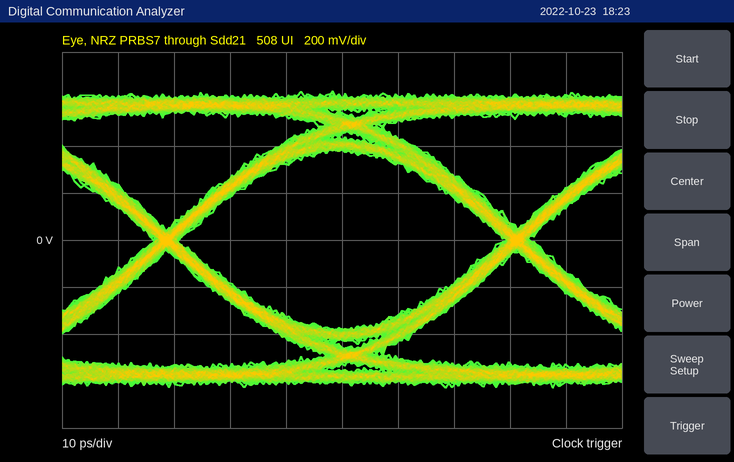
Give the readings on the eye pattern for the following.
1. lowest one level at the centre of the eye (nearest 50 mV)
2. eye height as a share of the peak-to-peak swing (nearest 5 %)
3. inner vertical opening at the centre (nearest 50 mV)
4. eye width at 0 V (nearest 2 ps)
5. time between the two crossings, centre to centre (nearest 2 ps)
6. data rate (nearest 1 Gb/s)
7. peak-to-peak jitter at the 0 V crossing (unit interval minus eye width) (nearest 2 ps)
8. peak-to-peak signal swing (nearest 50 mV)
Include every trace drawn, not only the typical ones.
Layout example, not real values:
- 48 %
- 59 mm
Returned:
- 400 mV
- 60 %
- 750 mV
- 58 ps
- 62 ps
- 16 Gb/s
- 4 ps
- 1.25 V
